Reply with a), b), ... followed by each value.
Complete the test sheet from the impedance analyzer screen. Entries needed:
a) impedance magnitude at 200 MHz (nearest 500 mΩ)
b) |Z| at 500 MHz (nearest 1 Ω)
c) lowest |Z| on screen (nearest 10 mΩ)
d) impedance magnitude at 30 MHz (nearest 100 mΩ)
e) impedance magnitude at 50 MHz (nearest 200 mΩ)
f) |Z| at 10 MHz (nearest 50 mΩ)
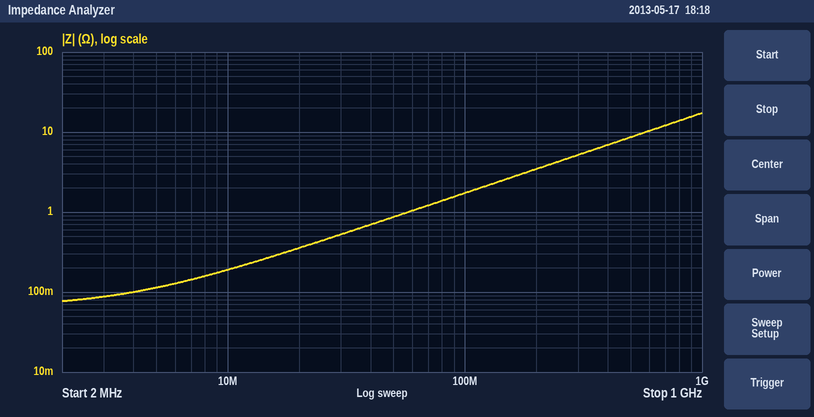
a) 3.5 Ω
b) 9 Ω
c) 80 mΩ
d) 500 mΩ
e) 800 mΩ
f) 200 mΩ
